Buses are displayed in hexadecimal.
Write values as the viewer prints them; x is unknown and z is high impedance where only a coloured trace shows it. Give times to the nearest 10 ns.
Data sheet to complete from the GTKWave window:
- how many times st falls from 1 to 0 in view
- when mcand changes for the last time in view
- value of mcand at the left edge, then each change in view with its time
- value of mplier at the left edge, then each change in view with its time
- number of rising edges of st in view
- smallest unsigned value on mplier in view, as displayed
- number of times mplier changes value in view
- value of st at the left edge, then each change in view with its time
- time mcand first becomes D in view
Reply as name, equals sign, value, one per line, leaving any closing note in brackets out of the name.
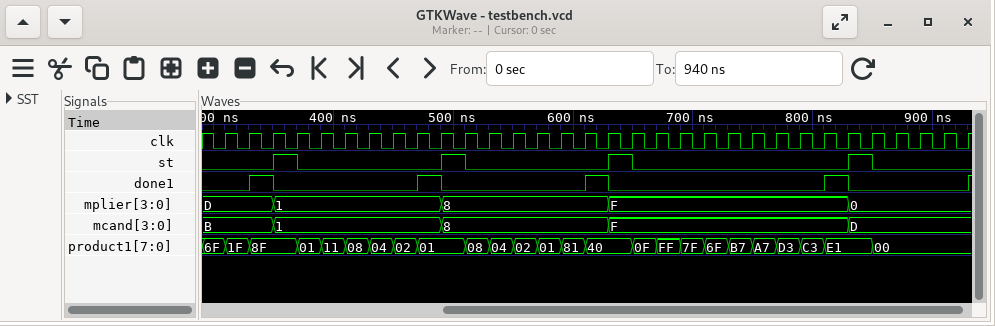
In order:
how many times st falls from 1 to 0 in view = 4
when mcand changes for the last time in view = 830 ns
value of mcand at the left edge, then each change in view with its time = B, 1 at 350 ns, 8 at 490 ns, F at 630 ns, D at 830 ns
value of mplier at the left edge, then each change in view with its time = D, 1 at 350 ns, 8 at 490 ns, F at 630 ns, 0 at 830 ns
number of rising edges of st in view = 4
smallest unsigned value on mplier in view, as displayed = 0
number of times mplier changes value in view = 4
value of st at the left edge, then each change in view with its time = 0, 1 at 350 ns, 0 at 370 ns, 1 at 490 ns, 0 at 510 ns, 1 at 630 ns, 0 at 650 ns, 1 at 830 ns, 0 at 850 ns
time mcand first becomes D in view = 830 ns
